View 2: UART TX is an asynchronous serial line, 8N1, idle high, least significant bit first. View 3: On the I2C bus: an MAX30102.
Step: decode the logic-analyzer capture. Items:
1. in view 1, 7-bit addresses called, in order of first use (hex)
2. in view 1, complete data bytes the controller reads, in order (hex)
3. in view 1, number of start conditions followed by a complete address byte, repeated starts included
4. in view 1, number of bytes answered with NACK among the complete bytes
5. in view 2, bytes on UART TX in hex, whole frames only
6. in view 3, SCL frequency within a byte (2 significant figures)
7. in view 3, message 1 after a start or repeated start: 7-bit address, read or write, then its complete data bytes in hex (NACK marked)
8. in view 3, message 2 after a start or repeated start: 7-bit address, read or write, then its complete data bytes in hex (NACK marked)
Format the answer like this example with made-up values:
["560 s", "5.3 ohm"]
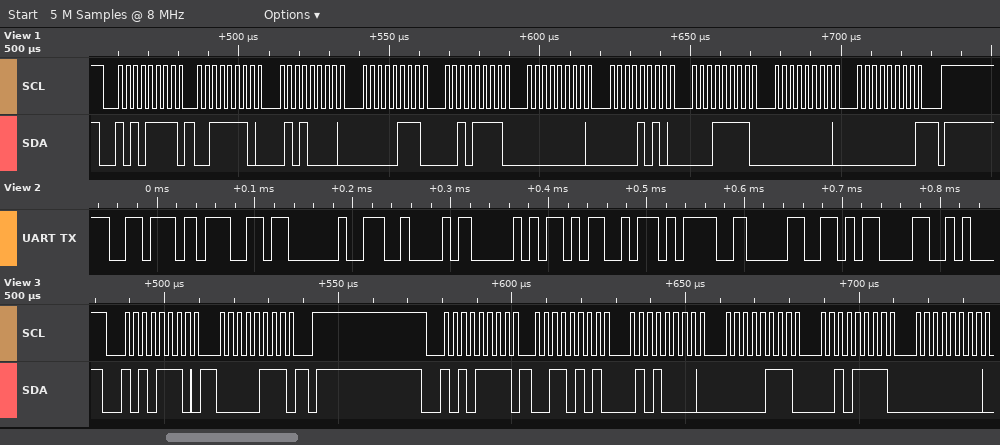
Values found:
["0x57", "3E 50 07 2F 00 0A 1F 00 00", "1", "1", "76 67 20 42 50 4D 3D 30 0D", "400 kHz", "0x57 write: 07", "0x57 read: 35 50 07 2F 00"]
